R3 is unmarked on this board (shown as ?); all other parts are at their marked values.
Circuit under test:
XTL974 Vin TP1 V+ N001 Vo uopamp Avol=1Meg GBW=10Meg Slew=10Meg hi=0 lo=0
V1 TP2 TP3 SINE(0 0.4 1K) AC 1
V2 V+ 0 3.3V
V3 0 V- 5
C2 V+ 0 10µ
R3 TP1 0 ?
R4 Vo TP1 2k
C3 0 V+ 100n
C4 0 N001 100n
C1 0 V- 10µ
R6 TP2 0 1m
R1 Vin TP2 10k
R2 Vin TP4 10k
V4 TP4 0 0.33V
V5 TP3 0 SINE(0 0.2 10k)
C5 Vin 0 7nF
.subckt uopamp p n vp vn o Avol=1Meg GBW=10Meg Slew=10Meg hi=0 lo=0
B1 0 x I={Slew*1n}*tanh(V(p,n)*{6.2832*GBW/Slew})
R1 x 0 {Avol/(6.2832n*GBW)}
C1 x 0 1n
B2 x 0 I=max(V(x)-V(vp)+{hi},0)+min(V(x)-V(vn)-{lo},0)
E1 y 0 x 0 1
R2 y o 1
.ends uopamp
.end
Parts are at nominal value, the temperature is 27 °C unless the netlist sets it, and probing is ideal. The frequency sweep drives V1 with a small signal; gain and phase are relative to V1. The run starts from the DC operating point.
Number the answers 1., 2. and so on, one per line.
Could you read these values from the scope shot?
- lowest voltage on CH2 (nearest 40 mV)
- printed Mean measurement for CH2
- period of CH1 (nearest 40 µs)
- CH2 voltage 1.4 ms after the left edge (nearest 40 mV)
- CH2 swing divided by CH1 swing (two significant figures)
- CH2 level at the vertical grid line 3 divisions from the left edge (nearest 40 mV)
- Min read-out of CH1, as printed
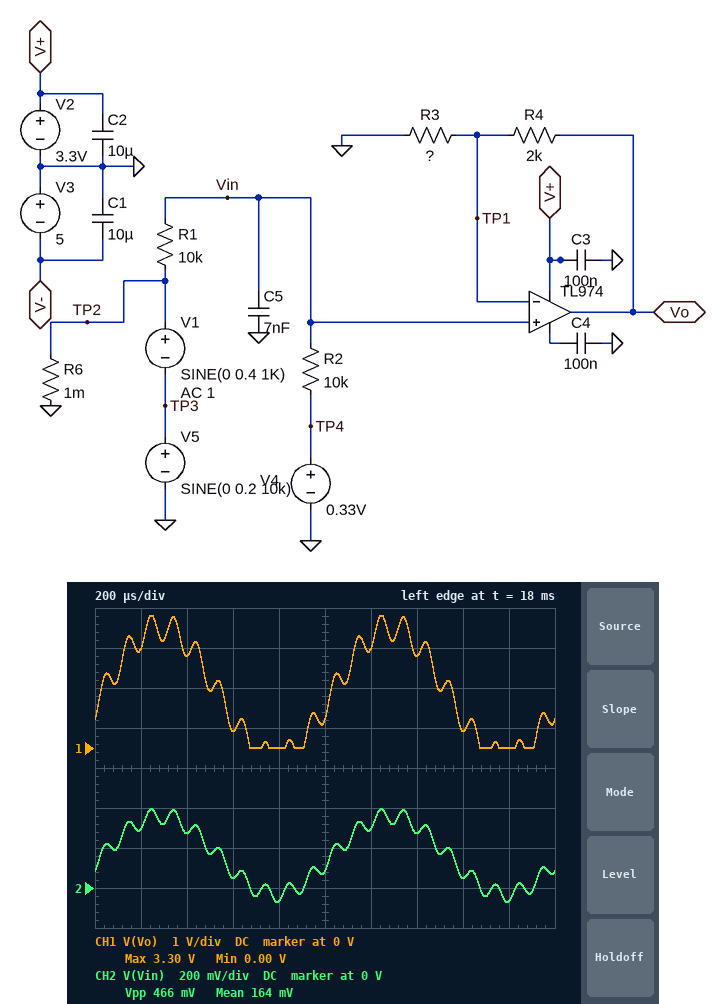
1. -80 mV
2. 164 mV
3. 1.00 ms
4. 280 mV
5. 0.14
6. 40 mV
7. 0.00 V
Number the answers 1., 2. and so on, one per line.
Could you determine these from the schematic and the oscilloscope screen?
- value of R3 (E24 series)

1. 270 Ω
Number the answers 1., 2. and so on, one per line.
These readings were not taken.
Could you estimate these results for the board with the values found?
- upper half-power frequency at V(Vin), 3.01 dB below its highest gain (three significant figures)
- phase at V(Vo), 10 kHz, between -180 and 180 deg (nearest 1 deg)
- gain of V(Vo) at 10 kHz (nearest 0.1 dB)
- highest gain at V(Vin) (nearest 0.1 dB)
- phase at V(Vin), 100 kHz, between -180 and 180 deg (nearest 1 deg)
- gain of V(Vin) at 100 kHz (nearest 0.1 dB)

1. 4.55 kHz
2. -66 deg
3. 4.8 dB
4. -6.0 dB
5. -87 deg
6. -32.9 dB
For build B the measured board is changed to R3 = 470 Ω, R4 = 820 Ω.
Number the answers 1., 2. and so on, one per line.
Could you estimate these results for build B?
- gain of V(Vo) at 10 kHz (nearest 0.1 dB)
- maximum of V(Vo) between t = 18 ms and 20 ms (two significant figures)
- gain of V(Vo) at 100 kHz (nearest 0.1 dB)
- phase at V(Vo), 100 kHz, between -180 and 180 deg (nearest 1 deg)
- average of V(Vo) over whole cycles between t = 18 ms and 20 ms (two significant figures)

1. -4.9 dB
2. 1.1 V
3. -24.1 dB
4. -89 deg
5. 470 mV
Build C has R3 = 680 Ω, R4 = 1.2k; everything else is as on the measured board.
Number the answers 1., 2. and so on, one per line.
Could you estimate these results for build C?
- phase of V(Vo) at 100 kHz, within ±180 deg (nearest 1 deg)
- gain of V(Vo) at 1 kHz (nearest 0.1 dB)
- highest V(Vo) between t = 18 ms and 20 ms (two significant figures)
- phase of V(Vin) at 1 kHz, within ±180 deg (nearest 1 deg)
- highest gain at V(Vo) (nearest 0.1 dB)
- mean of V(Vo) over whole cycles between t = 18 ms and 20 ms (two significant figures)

1. -89 deg
2. 2.6 dB
3. 1.1 V
4. -12 deg
5. 2.8 dB
6. 470 mV
